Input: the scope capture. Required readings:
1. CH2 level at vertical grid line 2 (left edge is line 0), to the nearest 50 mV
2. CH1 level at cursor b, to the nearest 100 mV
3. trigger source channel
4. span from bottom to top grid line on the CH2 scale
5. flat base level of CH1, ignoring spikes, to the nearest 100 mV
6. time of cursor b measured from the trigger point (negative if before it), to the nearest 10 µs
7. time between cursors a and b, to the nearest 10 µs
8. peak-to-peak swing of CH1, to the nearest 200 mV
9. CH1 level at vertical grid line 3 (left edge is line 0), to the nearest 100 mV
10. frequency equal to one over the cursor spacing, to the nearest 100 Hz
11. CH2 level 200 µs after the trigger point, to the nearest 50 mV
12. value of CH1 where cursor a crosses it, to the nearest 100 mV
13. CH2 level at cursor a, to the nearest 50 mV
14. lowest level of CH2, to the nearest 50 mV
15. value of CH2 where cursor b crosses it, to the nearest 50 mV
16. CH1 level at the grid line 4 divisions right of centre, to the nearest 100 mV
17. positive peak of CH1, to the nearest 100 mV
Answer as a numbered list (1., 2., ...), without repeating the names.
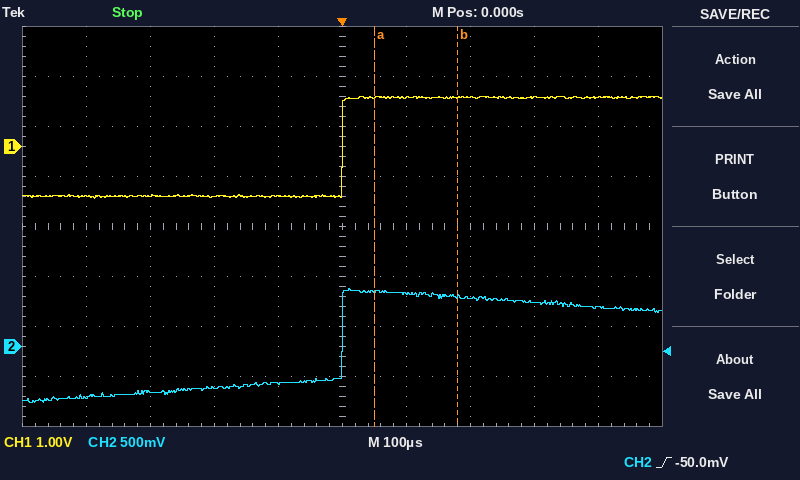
1. -450 mV
2. 1.0 V
3. CH2
4. 4 V
5. -1.0 V
6. +180 µs
7. 130 µs
8. 2.0 V
9. -1.0 V
10. 7.7 kHz
11. 500 mV
12. 1.0 V
13. 550 mV
14. -550 mV
15. 500 mV
16. 1.0 V
17. 1.0 V
